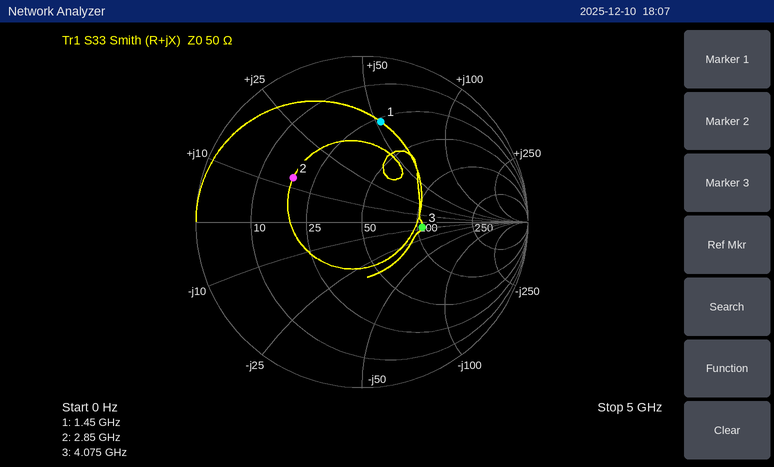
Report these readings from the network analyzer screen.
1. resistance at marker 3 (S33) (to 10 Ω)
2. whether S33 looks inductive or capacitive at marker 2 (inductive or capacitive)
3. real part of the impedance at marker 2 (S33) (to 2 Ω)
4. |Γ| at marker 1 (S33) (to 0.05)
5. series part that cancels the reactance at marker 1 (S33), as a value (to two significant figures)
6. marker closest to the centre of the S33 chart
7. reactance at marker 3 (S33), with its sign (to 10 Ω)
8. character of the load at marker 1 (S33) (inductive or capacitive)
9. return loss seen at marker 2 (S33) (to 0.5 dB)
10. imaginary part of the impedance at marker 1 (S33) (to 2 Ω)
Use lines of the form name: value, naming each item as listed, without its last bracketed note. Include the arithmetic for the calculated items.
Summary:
resistance at marker 3 (S33): 110 Ω
whether S33 looks inductive or capacitive at marker 2: inductive
real part of the impedance at marker 2 (S33): 18 Ω
|Γ| at marker 1 (S33): 0.60
series part that cancels the reactance at marker 1 (S33), as a value: C = 1/(2π × 1.45 GHz × 52 Ω) ≈ 2.1 pF
marker closest to the centre of the S33 chart: marker 3
reactance at marker 3 (S33), with its sign: -10 Ω
character of the load at marker 1 (S33): inductive
return loss seen at marker 2 (S33): 6.0 dB
imaginary part of the impedance at marker 1 (S33): +52 Ω
